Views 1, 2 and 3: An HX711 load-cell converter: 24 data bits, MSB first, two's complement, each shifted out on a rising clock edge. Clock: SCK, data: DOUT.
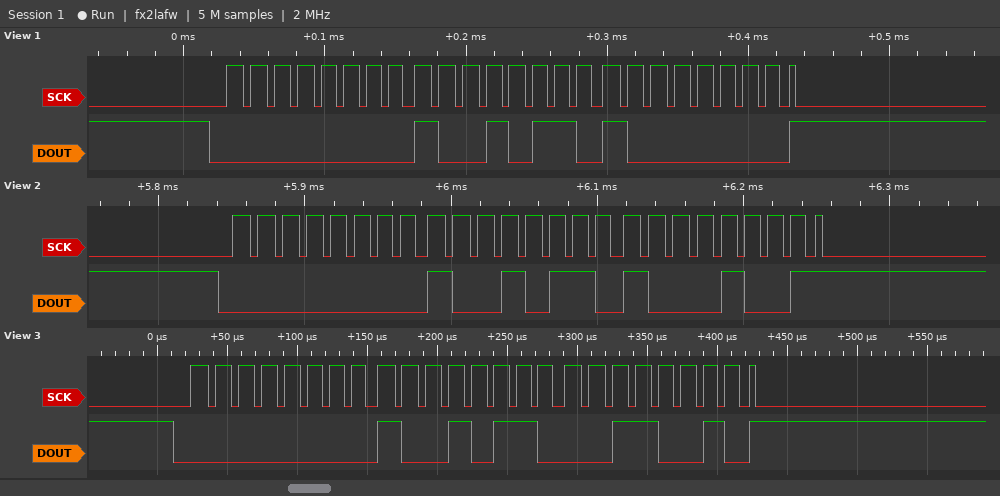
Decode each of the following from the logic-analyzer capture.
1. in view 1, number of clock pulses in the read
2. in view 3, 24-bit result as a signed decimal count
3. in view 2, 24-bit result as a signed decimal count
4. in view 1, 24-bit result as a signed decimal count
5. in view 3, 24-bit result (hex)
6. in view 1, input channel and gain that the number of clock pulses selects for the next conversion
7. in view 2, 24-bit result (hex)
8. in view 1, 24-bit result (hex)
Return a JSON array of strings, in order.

["25", "38450", "38537", "38528", "0x009632", "channel A, gain 128", "0x009689", "0x009680"]
